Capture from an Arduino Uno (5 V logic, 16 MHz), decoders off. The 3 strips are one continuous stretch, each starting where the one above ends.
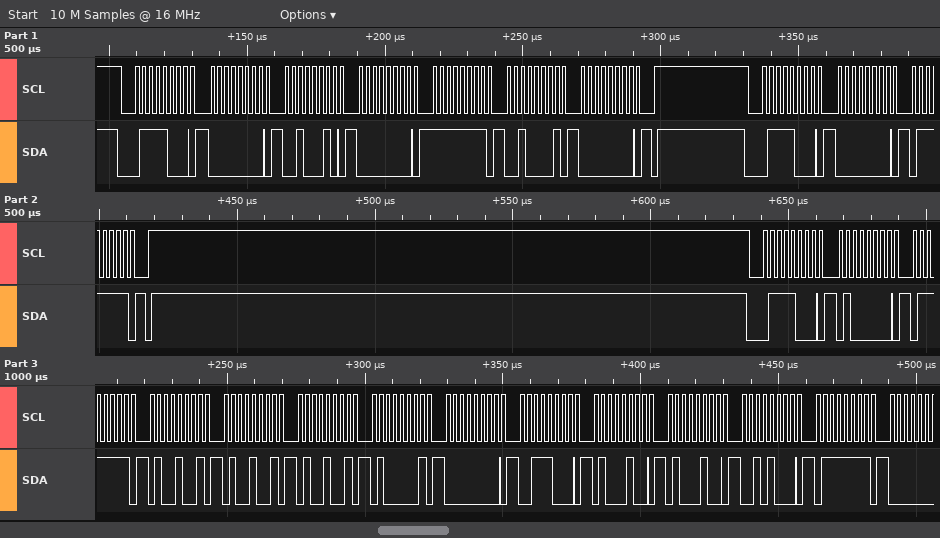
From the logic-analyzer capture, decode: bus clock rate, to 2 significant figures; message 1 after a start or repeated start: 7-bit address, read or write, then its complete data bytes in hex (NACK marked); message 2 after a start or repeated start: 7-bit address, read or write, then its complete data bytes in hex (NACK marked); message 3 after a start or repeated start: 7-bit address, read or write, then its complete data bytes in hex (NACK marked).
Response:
400 kHz
0x3C write: 00 22 00 FF 21 00
0x3C write: 00 7F
0x3C write: 40 7F 49 49 49 41 00 38 44 44 28 7F
